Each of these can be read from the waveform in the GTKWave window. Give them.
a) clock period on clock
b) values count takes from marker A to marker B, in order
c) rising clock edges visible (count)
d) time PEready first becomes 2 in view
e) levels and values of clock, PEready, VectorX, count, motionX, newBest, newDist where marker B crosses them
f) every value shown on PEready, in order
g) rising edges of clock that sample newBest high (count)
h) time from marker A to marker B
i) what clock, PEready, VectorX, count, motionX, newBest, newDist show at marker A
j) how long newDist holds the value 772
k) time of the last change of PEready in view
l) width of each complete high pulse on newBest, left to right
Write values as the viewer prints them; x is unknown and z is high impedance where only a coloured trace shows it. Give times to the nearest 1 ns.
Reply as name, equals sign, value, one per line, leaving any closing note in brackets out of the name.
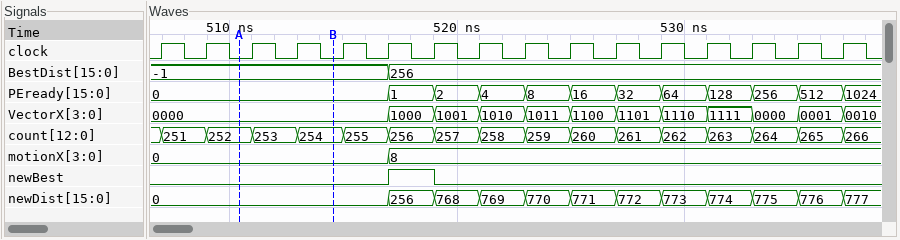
clock period on clock = 2 ns
values count takes from marker A to marker B, in order = 252, 253, 254
rising clock edges visible = 16
time PEready first becomes 2 in view = 519 ns
levels and values of clock, PEready, VectorX, count, motionX, newBest, newDist where marker B crosses them = clock=0, PEready=0, VectorX=0000, count=254, motionX=0, newBest=0, newDist=0
every value shown on PEready, in order = 0, 1, 2, 4, 8, 16, 32, 64, 128, 256, 512, 1024
rising edges of clock that sample newBest high = 1
time from marker A to marker B = 4 ns
what clock, PEready, VectorX, count, motionX, newBest, newDist show at marker A = clock=0, PEready=0, VectorX=0000, count=252, motionX=0, newBest=0, newDist=0
how long newDist holds the value 772 = 2 ns
time of the last change of PEready in view = 537 ns
width of each complete high pulse on newBest, left to right = 2 ns
